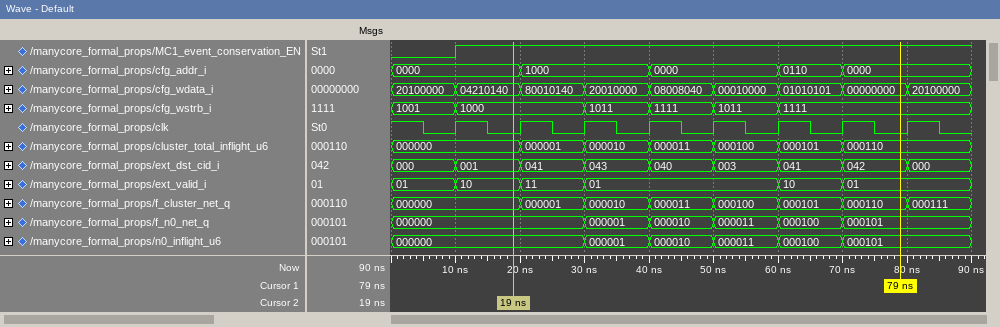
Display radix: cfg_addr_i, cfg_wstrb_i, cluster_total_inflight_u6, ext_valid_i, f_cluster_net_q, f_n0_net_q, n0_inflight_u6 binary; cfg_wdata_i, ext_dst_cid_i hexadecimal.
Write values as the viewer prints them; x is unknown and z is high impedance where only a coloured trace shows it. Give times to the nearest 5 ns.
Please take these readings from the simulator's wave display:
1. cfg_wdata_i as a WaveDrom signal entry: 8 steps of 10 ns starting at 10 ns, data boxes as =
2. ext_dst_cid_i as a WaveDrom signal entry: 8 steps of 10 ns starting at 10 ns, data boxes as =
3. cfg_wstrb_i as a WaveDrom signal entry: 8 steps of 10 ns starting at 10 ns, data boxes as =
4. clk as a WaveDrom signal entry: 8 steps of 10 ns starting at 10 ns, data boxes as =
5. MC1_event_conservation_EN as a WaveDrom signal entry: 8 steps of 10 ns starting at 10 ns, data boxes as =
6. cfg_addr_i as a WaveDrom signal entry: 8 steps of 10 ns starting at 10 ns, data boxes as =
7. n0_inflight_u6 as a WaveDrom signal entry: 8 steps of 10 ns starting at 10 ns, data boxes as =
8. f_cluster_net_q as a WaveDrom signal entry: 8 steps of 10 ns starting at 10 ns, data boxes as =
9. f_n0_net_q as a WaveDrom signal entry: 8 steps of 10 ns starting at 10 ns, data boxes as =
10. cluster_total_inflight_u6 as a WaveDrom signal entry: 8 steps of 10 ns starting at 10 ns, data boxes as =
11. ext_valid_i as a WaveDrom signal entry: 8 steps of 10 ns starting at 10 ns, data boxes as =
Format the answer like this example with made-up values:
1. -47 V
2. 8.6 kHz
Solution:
1. {name: 'cfg_wdata_i', wave: '========', data: '04210140 80010140 20010000 08008040 00010000 01010101 00000000 20100000'}
2. {name: 'ext_dst_cid_i', wave: '========', data: '001 041 043 040 003 041 042 000'}
3. {name: 'cfg_wstrb_i', wave: '=.====..', data: '1000 1011 1111 1011 1111'}
4. {name: 'clk', wave: 'p.......'}
5. {name: 'MC1_event_conservation_EN', wave: '1.......'}
6. {name: 'cfg_addr_i', wave: '==.=.==.', data: '0000 1000 0000 0110 0000'}
7. {name: 'n0_inflight_u6', wave: '=.=====.', data: '000000 000001 000010 000011 000100 000101'}
8. {name: 'f_cluster_net_q', wave: '========', data: '000000 000001 000010 000011 000100 000101 000110 000111'}
9. {name: 'f_n0_net_q', wave: '=.=====.', data: '000000 000001 000010 000011 000100 000101'}
10. {name: 'cluster_total_inflight_u6', wave: '=======.', data: '000000 000001 000010 000011 000100 000101 000110'}
11. {name: 'ext_valid_i', wave: '===..==.', data: '10 11 01 10 01'}
